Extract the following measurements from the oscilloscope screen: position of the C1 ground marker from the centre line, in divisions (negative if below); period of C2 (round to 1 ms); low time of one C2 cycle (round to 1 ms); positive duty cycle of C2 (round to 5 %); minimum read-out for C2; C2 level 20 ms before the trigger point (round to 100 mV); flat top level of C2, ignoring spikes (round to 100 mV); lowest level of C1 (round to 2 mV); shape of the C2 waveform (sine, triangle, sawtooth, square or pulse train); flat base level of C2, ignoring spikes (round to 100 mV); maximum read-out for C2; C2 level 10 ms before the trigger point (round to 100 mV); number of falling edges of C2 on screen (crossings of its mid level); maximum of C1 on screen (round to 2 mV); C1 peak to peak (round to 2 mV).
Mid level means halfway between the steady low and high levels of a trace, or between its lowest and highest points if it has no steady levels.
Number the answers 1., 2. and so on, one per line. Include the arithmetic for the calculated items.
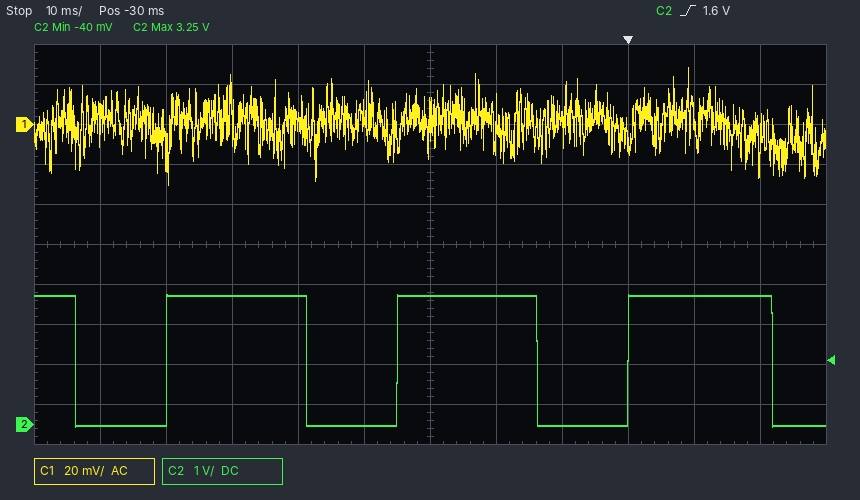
1. +3.0 div
2. 35 ms
3. 14 ms
4. 60 %
5. -40 mV
6. 3.2 V
7. 3.2 V
8. -30 mV
9. pulse train
10. 0.0 V
11. 3.25 V
12. 0.0 V
13. 4
14. 28 mV
15. 28 mV − (-30 mV) = 58 mV
